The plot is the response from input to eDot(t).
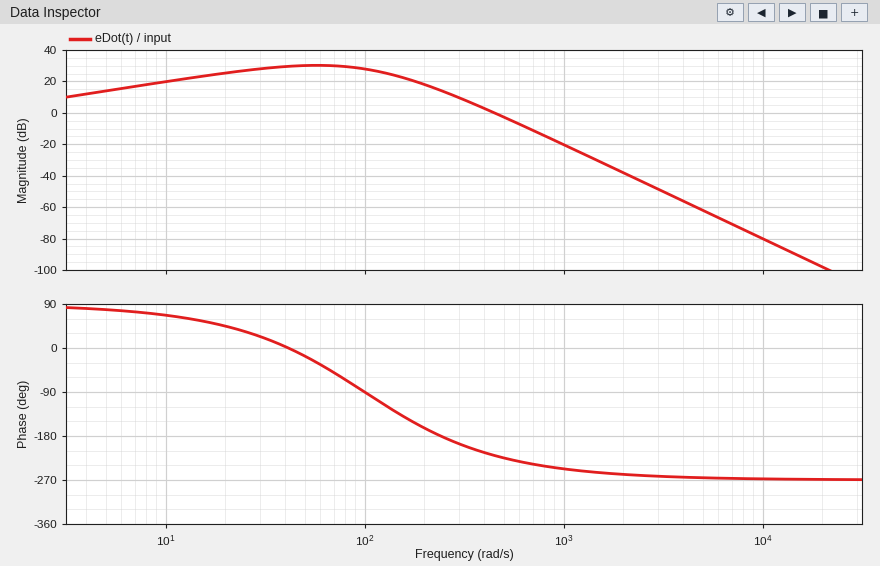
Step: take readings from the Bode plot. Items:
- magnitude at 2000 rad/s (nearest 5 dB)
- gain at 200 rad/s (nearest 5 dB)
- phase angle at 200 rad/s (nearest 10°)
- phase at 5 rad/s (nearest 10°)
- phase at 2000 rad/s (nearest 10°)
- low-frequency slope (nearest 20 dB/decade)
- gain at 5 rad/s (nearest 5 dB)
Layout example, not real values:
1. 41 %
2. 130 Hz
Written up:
1. -40 dB
2. 20 dB
3. -160°
4. 80°
5. -260°
6. 20 dB/decade
7. 15 dB
